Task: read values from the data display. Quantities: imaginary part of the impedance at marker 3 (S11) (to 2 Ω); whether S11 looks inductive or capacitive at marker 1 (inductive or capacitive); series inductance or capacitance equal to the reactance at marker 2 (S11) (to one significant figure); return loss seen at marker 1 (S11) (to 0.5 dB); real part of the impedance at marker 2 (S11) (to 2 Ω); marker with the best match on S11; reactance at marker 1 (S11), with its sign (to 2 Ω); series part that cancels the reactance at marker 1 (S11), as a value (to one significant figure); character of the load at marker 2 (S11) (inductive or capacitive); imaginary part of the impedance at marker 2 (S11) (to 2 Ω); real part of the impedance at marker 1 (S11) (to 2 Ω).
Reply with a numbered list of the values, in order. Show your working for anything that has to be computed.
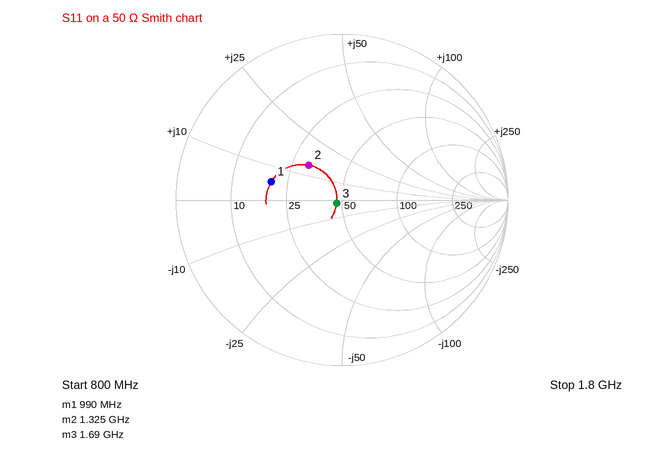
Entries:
1. -2 Ω
2. inductive
3. L = 14 Ω/(2π × 1.325 GHz) ≈ 2 nH
4. 7.0 dB
5. 30 Ω
6. marker 3
7. +6 Ω
8. C = 1/(2π × 990 MHz × 6 Ω) ≈ 26.8 pF, so 30 pF to one significant figure
9. inductive
10. +14 Ω
11. 20 Ω
